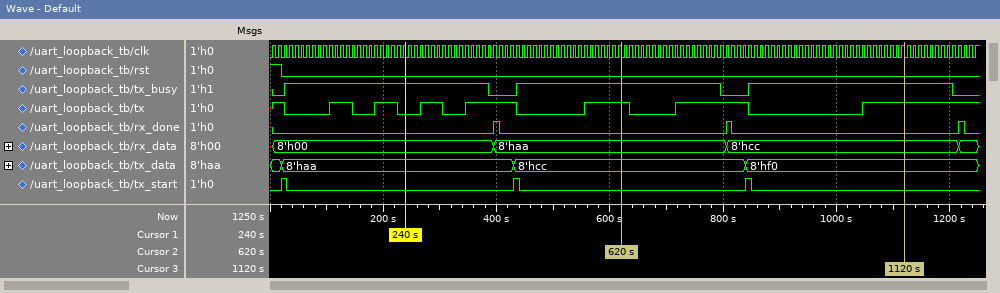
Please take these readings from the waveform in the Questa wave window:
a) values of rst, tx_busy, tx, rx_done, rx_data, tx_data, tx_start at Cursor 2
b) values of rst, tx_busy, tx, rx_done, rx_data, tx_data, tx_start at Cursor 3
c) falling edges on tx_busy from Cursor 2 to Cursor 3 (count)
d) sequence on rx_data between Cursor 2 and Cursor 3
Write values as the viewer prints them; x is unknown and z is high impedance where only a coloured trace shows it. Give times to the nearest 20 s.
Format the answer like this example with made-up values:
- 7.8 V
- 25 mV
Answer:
- rst=0, tx_busy=1, tx=1, rx_done=0, rx_data=8'haa, tx_data=8'hcc, tx_start=0
- rst=0, tx_busy=1, tx=1, rx_done=0, rx_data=8'hcc, tx_data=8'hf0, tx_start=0
- 1
- 8'haa, 8'hcc
